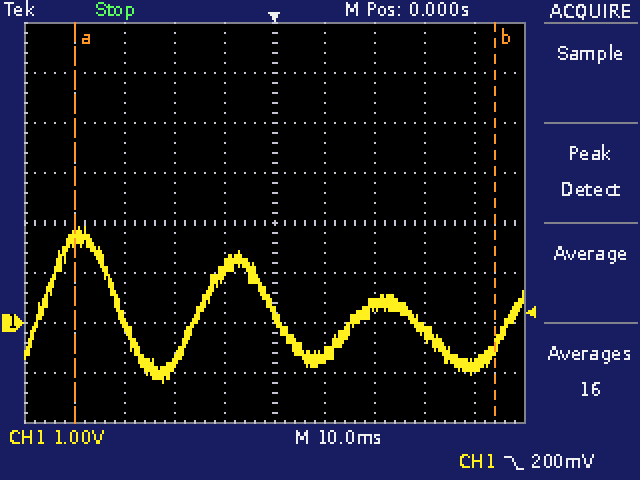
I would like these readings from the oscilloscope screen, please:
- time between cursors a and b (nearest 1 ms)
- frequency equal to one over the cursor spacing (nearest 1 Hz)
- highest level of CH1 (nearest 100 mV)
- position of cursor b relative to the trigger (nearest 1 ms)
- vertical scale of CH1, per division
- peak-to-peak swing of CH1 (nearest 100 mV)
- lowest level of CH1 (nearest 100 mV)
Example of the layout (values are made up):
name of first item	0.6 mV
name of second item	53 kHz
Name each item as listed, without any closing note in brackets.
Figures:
time between cursors a and b	84 ms
frequency equal to one over the cursor spacing	12 Hz
highest level of CH1	1.9 V
position of cursor b relative to the trigger	+44 ms
vertical scale of CH1, per division	1 V
peak-to-peak swing of CH1	3.1 V
lowest level of CH1	-1.2 V
